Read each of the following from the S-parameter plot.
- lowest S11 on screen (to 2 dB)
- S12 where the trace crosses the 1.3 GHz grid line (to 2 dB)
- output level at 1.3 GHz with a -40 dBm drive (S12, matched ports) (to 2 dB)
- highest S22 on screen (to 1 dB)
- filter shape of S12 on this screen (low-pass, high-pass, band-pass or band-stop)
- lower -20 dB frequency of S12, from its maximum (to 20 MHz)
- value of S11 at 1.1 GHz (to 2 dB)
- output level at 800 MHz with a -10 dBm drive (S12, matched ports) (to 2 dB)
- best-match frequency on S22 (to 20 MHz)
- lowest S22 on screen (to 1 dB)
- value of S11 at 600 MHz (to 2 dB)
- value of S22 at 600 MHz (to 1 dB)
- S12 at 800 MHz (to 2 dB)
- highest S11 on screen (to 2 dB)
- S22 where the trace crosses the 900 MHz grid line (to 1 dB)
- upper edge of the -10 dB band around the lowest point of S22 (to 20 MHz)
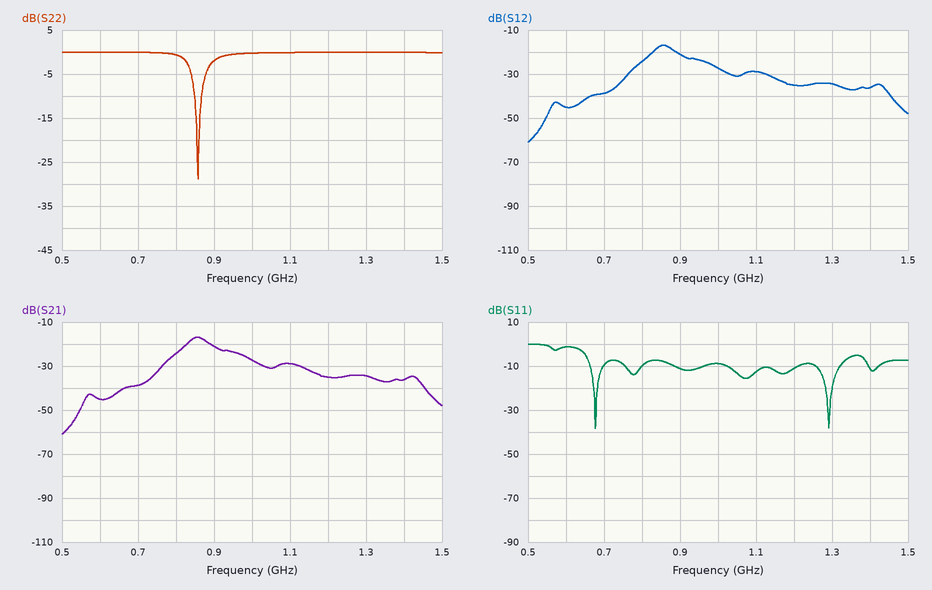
-38 dB
-34 dB
-74 dBm
0 dB
band-pass
720 MHz
-12 dB
-34 dBm
860 MHz
-29 dB
-2 dB
0 dB
-24 dB
0 dB
-2 dB
860 MHz
